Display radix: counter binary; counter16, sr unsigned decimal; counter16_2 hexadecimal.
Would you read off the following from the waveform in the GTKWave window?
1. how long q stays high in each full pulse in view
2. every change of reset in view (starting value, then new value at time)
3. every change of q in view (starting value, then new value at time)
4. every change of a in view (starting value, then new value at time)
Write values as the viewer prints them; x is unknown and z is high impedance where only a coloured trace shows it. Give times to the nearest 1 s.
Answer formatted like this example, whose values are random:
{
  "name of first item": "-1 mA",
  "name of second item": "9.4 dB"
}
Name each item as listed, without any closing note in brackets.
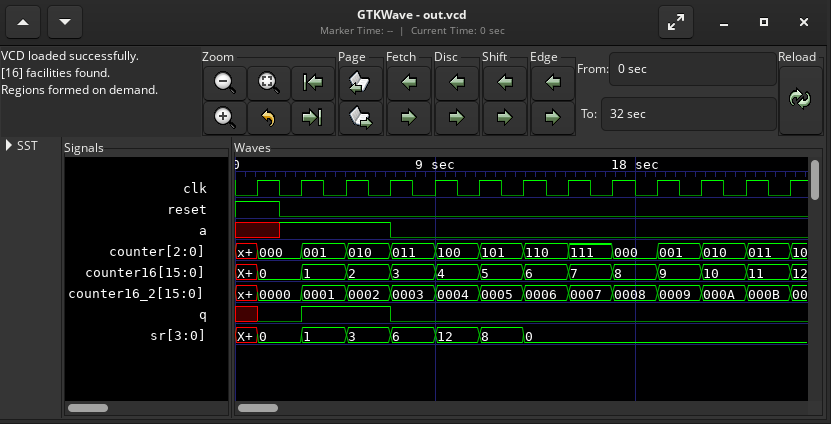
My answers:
{
  "how long q stays high in each full pulse in view": "4 s",
  "every change of reset in view": "1, 0 at 2 s",
  "every change of q in view": "x, 0 at 1 s, 1 at 3 s, 0 at 7 s",
  "every change of a in view": "x, 1 at 2 s, 0 at 7 s"
}
